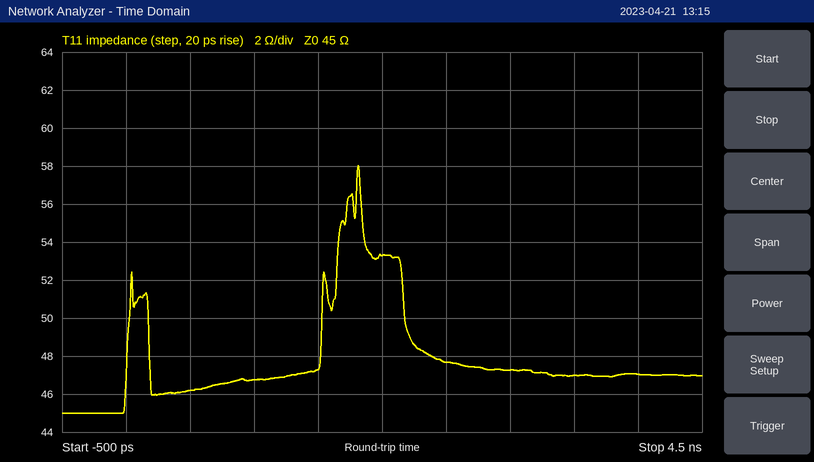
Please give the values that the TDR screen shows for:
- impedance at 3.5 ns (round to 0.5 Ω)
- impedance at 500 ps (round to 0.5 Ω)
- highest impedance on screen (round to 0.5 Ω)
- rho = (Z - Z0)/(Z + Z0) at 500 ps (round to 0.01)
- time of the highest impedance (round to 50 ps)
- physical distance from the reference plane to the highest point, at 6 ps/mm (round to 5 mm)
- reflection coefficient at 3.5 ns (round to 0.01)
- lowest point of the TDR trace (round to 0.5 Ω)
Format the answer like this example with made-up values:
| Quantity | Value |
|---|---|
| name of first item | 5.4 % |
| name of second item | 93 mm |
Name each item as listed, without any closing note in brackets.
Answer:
| Quantity | Value |
|---|---|
| impedance at 3.5 ns | 47.0 Ω |
| impedance at 500 ps | 46.0 Ω |
| highest impedance on screen | 58.0 Ω |
| rho = (Z - Z0)/(Z + Z0) at 500 ps | +0.01 |
| time of the highest impedance | 1.80 ns |
| physical distance from the reference plane to the highest point, at 6 ps/mm | 150 mm |
| reflection coefficient at 3.5 ns | +0.02 |
| lowest point of the TDR trace | 45.0 Ω |
